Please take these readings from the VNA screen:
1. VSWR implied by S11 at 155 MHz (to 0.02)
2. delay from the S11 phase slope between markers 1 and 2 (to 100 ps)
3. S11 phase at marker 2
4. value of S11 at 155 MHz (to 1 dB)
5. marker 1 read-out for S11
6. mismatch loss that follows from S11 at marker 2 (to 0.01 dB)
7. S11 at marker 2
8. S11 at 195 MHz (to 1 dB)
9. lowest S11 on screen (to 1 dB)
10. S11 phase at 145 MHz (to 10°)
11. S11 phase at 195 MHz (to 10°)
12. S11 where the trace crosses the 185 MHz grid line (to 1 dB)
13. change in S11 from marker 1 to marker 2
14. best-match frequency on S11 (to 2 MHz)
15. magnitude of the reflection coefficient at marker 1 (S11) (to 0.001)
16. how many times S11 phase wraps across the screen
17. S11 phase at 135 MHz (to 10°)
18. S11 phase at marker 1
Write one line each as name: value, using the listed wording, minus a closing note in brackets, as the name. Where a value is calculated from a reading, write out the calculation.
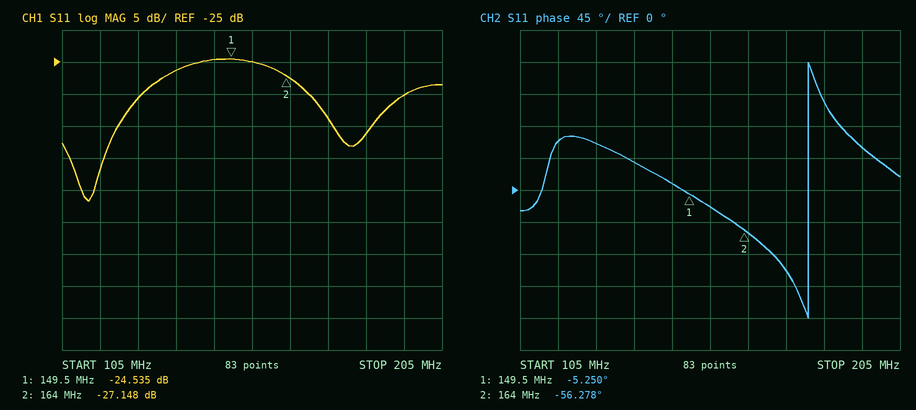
VSWR implied by S11 at 155 MHz: |Γ| = 10^(-25/20) = 0.0562; VSWR = (1 + 0.0562)/(1 − 0.0562) ≈ 1.12
delay from the S11 phase slope between markers 1 and 2: −(-56.278° − (-5.25°))/(360° × 14.5 MHz) ≈ 9.8 ns
S11 phase at marker 2: -56.278°
value of S11 at 155 MHz: -25 dB
marker 1 read-out for S11: -24.535 dB
mismatch loss that follows from S11 at marker 2: −10 log10(1 − 10^(-27.148/10)) ≈ 0.01 dB
S11 at marker 2: -27.148 dB
S11 at 195 MHz: -30 dB
lowest S11 on screen: -47 dB
S11 phase at 145 MHz: 10°
S11 phase at 195 MHz: 60°
S11 where the trace crosses the 185 MHz grid line: -36 dB
change in S11 from marker 1 to marker 2: -27.148 − (-24.535) = -2.613 dB
best-match frequency on S11: 112 MHz
magnitude of the reflection coefficient at marker 1 (S11): 10^(-24.535/20) ≈ 0.059
how many times S11 phase wraps across the screen: 1
S11 phase at 135 MHz: 40°
S11 phase at marker 1: -5.250°
